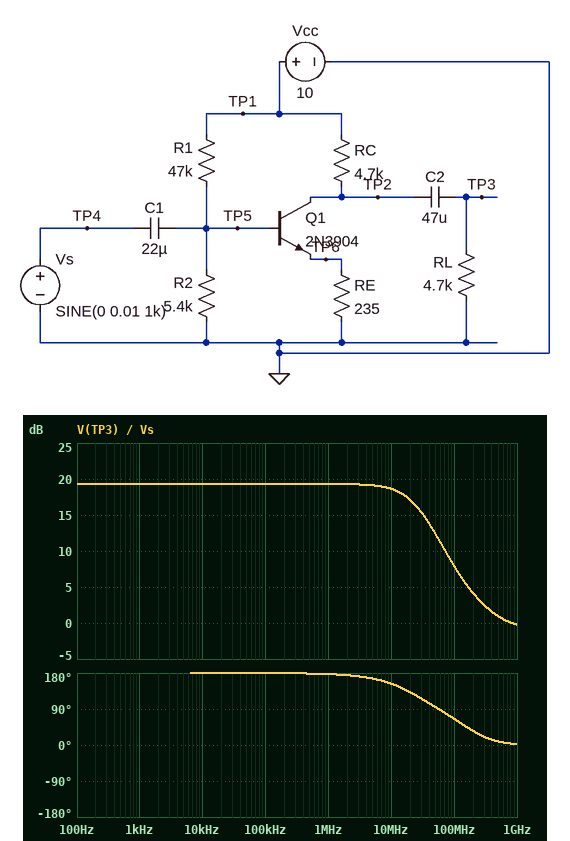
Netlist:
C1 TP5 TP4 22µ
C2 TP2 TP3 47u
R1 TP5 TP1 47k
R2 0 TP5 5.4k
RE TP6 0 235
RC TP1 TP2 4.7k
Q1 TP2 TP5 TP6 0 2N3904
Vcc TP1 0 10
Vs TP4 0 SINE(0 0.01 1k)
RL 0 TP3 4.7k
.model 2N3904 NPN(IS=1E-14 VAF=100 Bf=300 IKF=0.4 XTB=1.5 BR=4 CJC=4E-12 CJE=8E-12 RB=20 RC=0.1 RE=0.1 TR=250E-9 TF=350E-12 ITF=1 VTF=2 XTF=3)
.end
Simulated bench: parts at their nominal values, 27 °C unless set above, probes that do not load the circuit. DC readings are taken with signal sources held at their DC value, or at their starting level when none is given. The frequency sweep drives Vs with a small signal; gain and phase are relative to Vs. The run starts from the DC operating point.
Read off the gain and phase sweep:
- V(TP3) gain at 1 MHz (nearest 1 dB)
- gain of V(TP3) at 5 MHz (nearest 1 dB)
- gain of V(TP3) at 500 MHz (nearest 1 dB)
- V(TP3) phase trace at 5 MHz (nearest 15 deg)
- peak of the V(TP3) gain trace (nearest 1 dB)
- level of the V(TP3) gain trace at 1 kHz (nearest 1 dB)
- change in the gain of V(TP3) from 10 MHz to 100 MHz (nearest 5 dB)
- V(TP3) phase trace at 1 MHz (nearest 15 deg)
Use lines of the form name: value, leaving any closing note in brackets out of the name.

V(TP3) gain at 1 MHz: 19 dB
gain of V(TP3) at 5 MHz: 19 dB
gain of V(TP3) at 500 MHz: 1 dB
V(TP3) phase trace at 5 MHz: 165 deg
peak of the V(TP3) gain trace: 19 dB
level of the V(TP3) gain trace at 1 kHz: 19 dB
change in the gain of V(TP3) from 10 MHz to 100 MHz: -10 dB
V(TP3) phase trace at 1 MHz: 180 deg
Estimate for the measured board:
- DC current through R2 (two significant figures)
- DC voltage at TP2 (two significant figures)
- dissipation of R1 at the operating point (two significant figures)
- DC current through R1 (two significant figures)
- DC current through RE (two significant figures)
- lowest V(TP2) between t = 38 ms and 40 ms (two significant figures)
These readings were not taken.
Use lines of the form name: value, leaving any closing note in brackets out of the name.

DC current through R2: 190 µA
DC voltage at TP2: 3.2 V
dissipation of R1 at the operating point: 1.7 mW
DC current through R1: 190 µA
DC current through RE: 1.5 mA
lowest V(TP2) between t = 38 ms and 40 ms: 3.1 V
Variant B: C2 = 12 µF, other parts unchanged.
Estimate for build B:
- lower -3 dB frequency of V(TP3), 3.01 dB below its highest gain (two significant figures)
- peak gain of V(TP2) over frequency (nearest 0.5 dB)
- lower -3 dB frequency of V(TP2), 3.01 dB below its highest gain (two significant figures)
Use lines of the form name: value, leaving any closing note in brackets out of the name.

lower -3 dB frequency of V(TP3), 3.01 dB below its highest gain: 2.3 Hz
peak gain of V(TP2) over frequency: 20.0 dB
lower -3 dB frequency of V(TP2), 3.01 dB below its highest gain: 760 mHz
